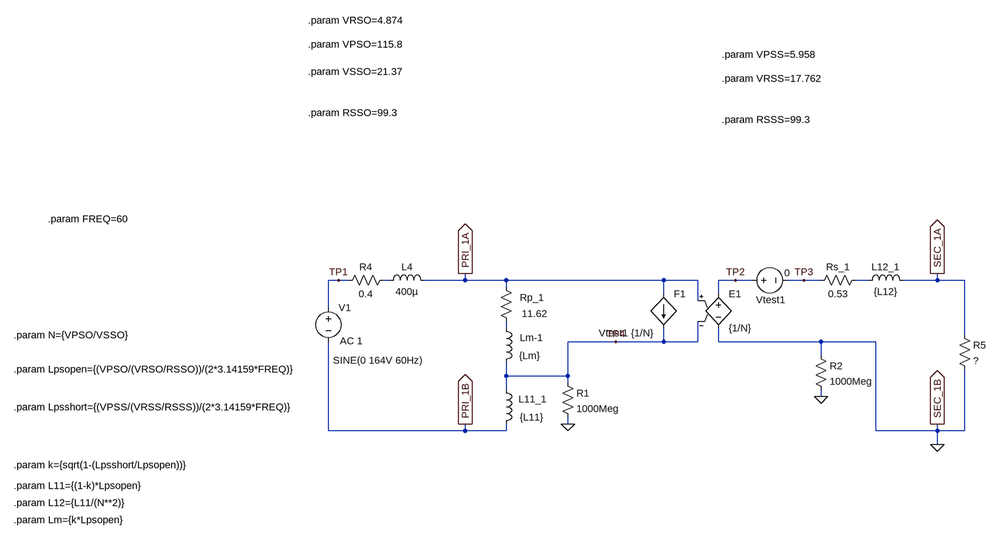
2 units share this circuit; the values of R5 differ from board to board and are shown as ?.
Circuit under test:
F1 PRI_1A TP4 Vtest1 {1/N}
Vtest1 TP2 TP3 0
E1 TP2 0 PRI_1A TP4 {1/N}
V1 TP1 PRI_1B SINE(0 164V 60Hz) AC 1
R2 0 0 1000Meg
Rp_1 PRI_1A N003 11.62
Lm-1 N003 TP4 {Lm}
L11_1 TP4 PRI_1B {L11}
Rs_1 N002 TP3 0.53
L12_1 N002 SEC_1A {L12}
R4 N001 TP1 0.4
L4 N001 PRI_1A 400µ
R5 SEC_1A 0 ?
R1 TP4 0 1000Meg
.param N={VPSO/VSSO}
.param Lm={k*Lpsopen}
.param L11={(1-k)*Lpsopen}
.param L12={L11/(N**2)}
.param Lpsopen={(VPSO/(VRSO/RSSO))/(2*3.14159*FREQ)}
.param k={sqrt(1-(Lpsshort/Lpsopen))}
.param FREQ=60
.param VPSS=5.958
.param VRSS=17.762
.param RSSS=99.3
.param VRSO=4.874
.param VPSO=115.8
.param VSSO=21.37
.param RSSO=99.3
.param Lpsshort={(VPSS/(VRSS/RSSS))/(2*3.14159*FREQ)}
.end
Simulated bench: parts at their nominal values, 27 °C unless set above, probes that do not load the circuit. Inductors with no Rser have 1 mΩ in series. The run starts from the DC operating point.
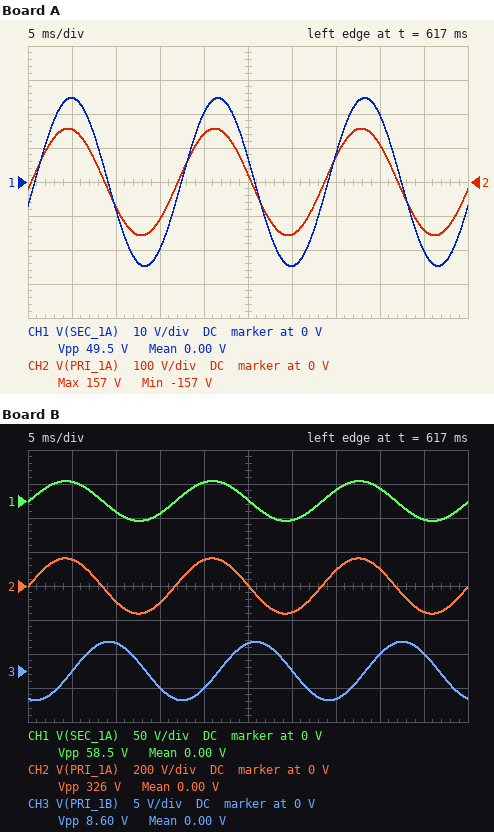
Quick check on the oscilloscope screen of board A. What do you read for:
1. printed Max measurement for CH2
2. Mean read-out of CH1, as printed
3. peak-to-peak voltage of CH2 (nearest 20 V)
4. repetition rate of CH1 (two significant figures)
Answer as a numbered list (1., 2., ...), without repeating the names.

1. 157 V
2. 0.00 V
3. 320 V
4. 60 Hz
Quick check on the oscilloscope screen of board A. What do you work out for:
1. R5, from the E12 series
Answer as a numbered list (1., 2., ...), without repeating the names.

1. 3.3 Ω
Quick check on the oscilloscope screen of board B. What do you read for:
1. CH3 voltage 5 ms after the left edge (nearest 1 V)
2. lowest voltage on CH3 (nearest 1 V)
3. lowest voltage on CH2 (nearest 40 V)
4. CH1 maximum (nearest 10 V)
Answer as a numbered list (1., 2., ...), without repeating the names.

1. 0 V
2. -4 V
3. -160 V
4. 30 V
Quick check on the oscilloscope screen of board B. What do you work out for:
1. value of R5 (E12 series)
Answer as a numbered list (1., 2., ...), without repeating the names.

1. 22 Ω
